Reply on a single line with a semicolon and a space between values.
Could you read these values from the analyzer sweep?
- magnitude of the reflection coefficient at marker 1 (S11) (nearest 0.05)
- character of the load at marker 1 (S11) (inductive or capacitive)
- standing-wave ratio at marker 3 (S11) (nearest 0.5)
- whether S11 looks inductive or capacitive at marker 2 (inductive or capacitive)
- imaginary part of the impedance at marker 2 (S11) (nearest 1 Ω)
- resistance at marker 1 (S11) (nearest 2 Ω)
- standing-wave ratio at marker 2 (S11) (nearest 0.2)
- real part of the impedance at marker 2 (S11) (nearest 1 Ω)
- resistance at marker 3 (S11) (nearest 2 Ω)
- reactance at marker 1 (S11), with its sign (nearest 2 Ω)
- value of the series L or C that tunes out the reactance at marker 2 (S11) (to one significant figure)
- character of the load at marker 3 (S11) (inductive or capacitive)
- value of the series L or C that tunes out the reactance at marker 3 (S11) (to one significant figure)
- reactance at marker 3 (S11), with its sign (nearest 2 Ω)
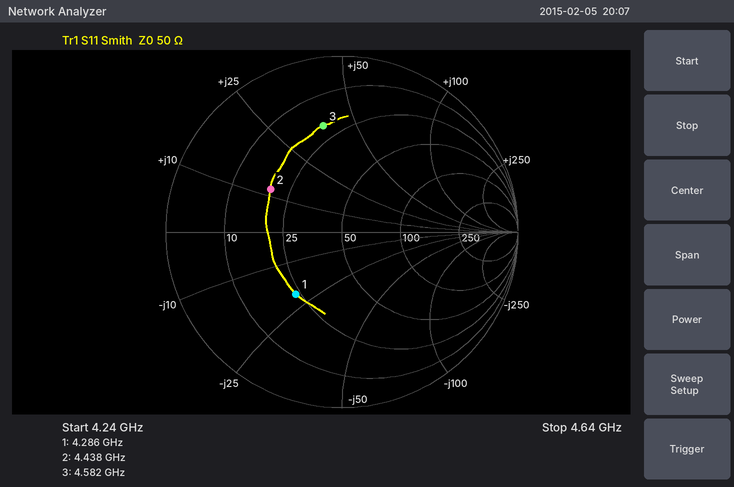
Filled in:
0.45; capacitive; 4.0; inductive; +12 Ω; 24 Ω; 2.8; 19 Ω; 20 Ω; -20 Ω; 3 pF; inductive; 900 fF; +38 Ω
